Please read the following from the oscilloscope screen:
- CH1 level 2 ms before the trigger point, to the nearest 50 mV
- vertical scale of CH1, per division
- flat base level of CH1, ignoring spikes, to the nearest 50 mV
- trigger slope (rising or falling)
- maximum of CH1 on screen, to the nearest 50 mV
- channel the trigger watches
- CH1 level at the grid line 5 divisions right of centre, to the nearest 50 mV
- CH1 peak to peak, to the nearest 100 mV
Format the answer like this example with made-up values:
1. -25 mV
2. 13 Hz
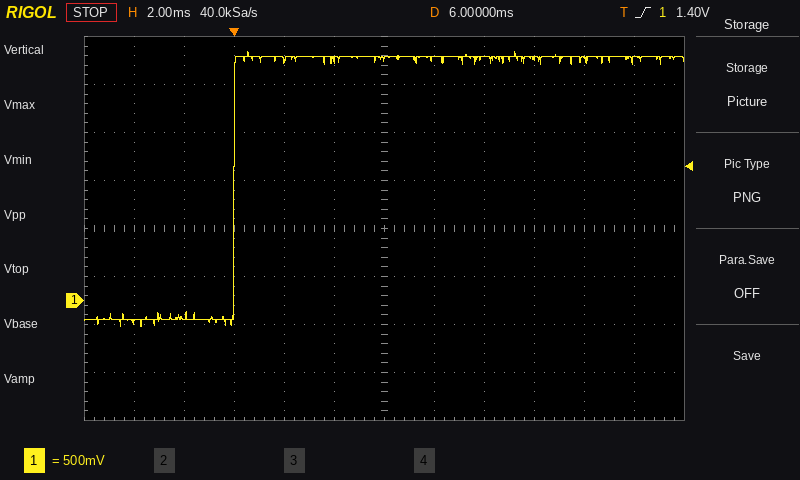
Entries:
1. -150 mV
2. 500 mV
3. -200 mV
4. rising
5. 2.60 V
6. CH1
7. 2.50 V
8. 2.90 V
